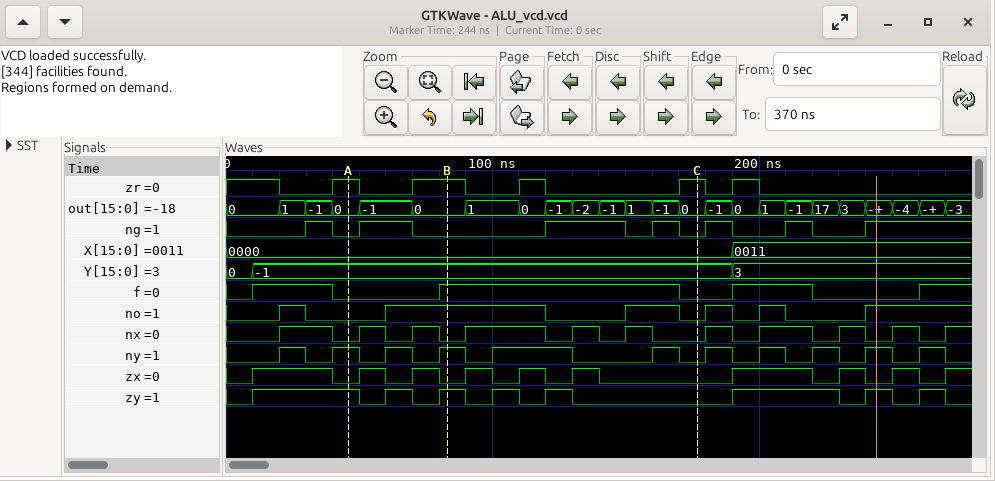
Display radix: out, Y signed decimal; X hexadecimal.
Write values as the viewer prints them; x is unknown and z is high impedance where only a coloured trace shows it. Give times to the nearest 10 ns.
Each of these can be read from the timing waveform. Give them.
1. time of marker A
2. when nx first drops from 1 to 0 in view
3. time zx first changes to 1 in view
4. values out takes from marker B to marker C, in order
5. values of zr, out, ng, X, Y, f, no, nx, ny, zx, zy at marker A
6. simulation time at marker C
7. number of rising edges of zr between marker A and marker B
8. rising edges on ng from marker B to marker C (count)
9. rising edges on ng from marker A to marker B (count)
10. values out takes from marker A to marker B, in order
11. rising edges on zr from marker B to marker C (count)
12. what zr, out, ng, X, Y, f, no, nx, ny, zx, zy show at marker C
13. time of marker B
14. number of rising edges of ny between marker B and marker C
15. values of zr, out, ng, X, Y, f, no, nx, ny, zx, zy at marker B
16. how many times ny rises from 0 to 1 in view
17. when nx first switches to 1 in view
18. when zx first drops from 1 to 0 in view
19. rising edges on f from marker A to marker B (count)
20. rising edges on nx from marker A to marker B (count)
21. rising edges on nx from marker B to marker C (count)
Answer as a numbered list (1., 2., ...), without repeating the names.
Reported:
1. 50 ns
2. 40 ns
3. 10 ns
4. 0, 1, 0, -1, -2, -1, 1, -1, 0
5. zr=1, out=0, ng=0, X=0000, Y=-1, f=0, no=0, nx=0, ny=1, zx=0, zy=1
6. 180 ns
7. 1
8. 2
9. 1
10. 0, -1, 0
11. 2
12. zr=1, out=0, ng=0, X=0000, Y=-1, f=0, no=0, nx=0, ny=0, zx=0, zy=0
13. 80 ns
14. 2
15. zr=1, out=0, ng=0, X=0000, Y=-1, f=1, no=1, nx=0, ny=1, zx=0, zy=1
16. 11
17. 20 ns
18. 40 ns
19. 1
20. 2
21. 3
